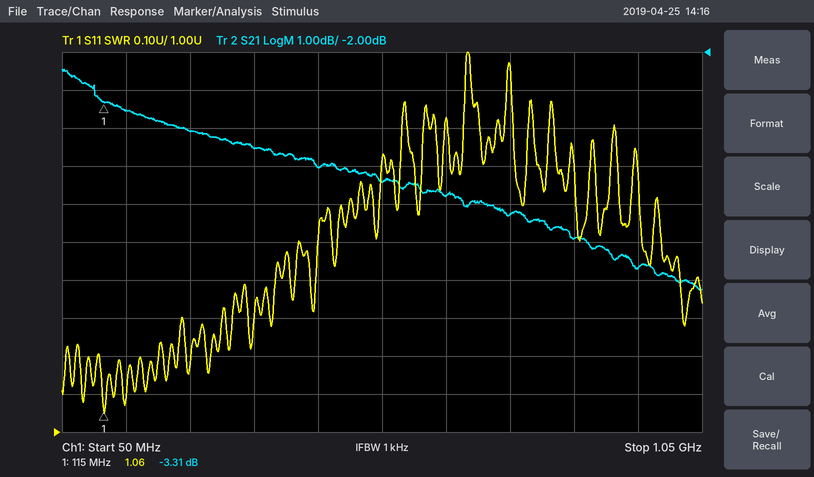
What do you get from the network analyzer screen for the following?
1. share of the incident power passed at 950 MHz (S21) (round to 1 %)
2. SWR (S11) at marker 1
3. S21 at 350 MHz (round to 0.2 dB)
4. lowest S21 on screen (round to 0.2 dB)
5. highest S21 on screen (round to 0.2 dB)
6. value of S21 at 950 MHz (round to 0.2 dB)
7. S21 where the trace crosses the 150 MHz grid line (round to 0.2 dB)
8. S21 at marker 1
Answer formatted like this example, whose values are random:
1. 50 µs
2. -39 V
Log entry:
1. 17 %
2. 1.06
3. -4.6 dB
4. -8.2 dB
5. -2.4 dB
6. -7.6 dB
7. -3.6 dB
8. -3.31 dB
